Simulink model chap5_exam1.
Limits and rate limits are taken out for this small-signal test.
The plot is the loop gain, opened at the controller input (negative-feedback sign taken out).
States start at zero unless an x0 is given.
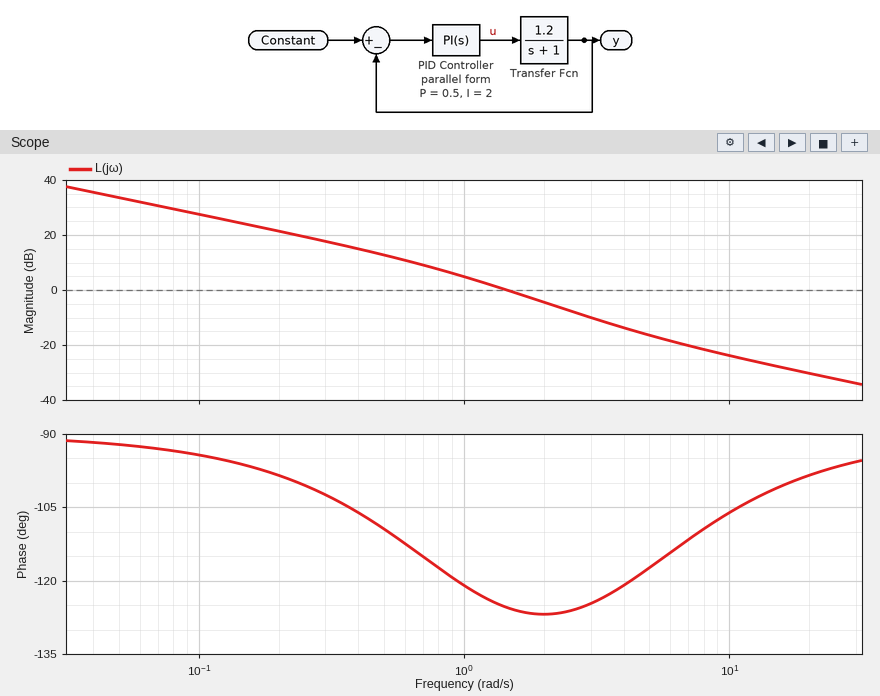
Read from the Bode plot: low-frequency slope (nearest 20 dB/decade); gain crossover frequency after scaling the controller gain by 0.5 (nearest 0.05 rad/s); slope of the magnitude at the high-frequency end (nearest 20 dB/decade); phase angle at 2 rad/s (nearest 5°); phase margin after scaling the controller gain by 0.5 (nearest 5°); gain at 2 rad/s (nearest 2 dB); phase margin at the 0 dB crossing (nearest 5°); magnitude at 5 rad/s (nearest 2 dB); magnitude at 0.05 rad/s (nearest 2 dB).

-20 dB/decade
0.90 rad/s
-20 dB/decade
-125°
60°
-4 dB
55°
-16 dB
34 dB
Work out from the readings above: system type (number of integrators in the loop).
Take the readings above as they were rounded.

1
